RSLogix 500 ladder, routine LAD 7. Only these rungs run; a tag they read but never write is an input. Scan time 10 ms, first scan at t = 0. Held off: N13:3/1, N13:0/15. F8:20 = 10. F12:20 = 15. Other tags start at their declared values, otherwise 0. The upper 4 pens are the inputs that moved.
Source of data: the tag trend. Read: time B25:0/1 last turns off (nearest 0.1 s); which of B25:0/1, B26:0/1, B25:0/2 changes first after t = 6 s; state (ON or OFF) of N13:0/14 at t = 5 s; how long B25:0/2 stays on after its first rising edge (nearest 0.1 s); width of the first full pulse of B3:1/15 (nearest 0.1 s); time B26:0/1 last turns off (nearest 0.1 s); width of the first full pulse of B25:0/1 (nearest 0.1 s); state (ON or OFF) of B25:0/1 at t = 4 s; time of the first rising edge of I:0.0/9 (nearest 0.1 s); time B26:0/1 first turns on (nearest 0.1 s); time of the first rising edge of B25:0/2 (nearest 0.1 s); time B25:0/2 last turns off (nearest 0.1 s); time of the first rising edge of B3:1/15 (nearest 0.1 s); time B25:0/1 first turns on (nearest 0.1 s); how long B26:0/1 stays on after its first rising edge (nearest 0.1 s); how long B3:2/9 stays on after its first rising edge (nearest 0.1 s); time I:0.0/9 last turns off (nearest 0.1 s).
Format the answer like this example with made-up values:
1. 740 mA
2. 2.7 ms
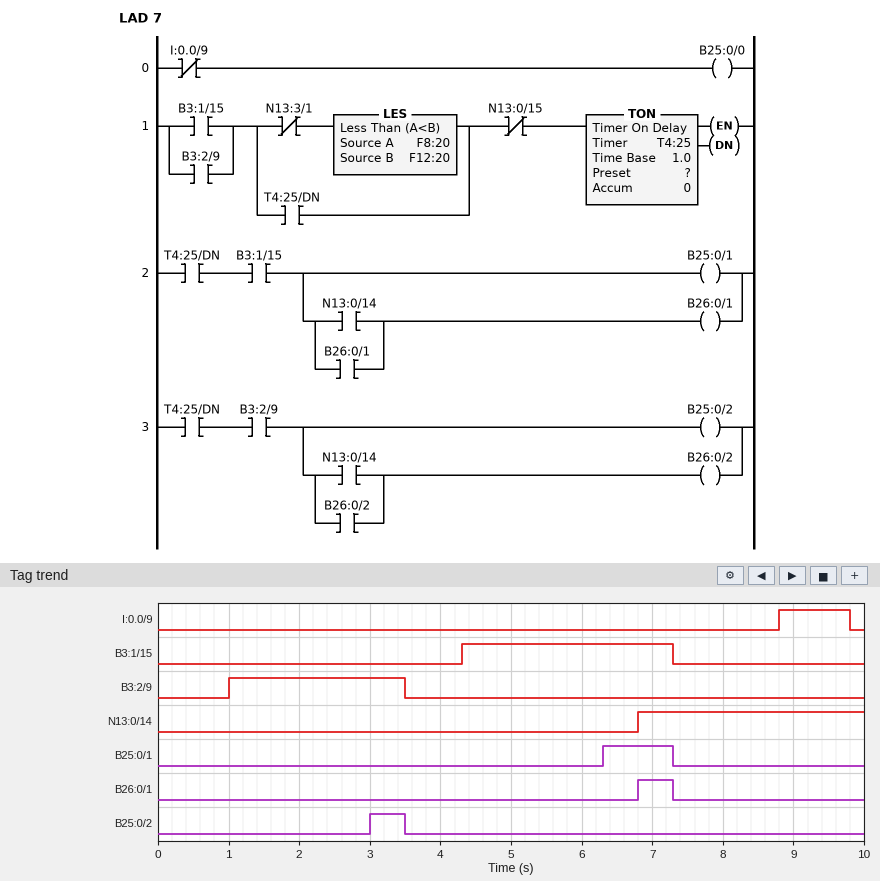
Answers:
1. 7.3 s
2. B25:0/1
3. OFF
4. 0.5 s
5. 3.0 s
6. 7.3 s
7. 1.0 s
8. OFF
9. 8.8 s
10. 6.8 s
11. 3.0 s
12. 3.5 s
13. 4.3 s
14. 6.3 s
15. 0.5 s
16. 2.5 s
17. 9.8 s
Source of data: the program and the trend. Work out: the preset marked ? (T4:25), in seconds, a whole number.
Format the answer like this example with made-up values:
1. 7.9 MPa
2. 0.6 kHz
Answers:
1. 2 s
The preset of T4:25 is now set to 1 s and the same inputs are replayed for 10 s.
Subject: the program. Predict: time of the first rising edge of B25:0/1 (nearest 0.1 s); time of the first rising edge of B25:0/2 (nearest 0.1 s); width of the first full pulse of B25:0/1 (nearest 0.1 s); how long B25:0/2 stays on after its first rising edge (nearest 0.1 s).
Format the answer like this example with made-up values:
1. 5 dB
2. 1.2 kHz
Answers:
1. 5.3 s
2. 2.0 s
3. 2.0 s
4. 1.5 s
